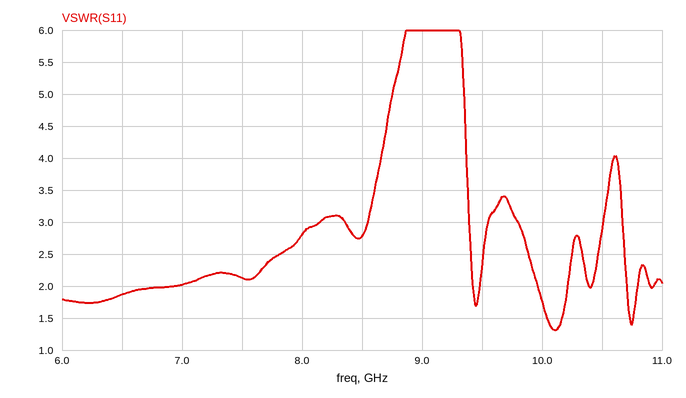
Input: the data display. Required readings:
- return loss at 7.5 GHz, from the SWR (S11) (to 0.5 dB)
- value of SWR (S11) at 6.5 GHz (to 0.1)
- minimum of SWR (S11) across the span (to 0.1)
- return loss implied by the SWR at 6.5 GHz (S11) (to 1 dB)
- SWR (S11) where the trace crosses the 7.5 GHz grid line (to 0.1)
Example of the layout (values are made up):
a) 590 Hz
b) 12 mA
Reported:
a) 9.0 dB
b) 1.9
c) 1.3
d) 10 dB
e) 2.1
